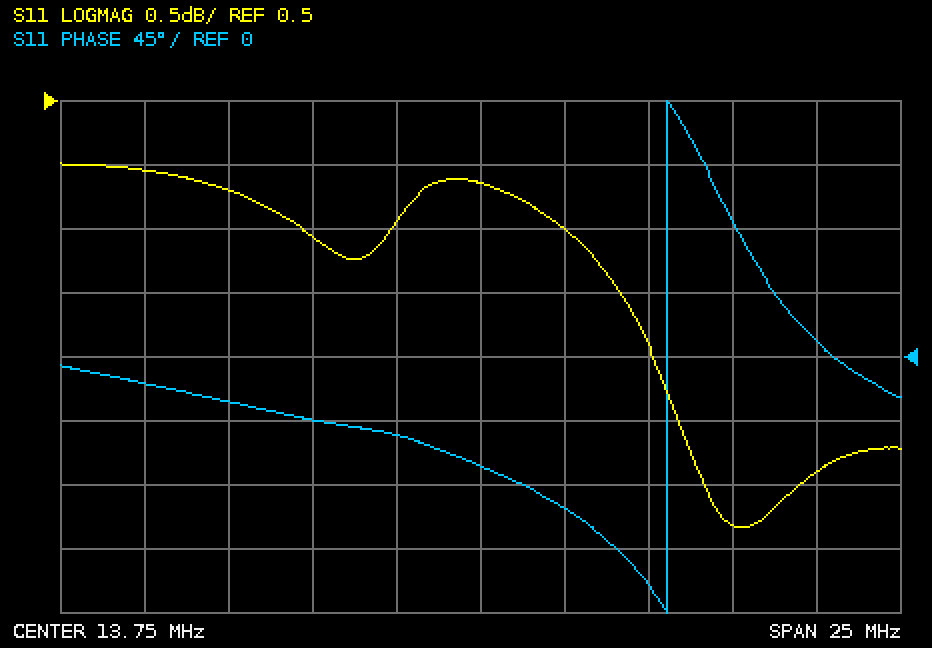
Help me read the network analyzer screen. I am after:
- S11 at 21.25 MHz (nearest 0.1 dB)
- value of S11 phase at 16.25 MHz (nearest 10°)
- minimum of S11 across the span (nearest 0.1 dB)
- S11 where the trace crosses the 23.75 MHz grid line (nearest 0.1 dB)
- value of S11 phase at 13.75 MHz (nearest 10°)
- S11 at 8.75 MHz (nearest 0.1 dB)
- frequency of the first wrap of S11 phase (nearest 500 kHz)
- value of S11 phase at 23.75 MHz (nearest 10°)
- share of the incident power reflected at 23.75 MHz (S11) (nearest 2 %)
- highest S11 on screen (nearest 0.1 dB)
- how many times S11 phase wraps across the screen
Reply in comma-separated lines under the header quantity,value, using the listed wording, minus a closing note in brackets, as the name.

quantity,value
S11 at 21.25 MHz,-2.8 dB
value of S11 phase at 16.25 MHz,-110°
minimum of S11 across the span,-2.8 dB
S11 where the trace crosses the 23.75 MHz grid line,-2.4 dB
value of S11 phase at 13.75 MHz,-80°
S11 at 8.75 MHz,-0.6 dB
frequency of the first wrap of S11 phase,19.5 MHz
value of S11 phase at 23.75 MHz,10°
share of the incident power reflected at 23.75 MHz (S11),58 %
highest S11 on screen,0.0 dB
how many times S11 phase wraps across the screen,1
